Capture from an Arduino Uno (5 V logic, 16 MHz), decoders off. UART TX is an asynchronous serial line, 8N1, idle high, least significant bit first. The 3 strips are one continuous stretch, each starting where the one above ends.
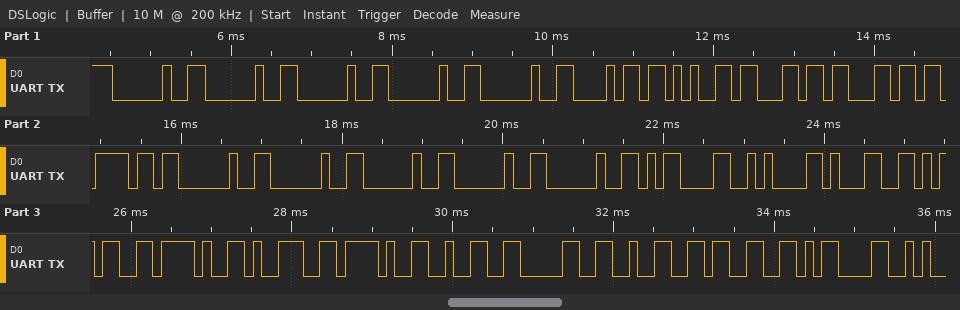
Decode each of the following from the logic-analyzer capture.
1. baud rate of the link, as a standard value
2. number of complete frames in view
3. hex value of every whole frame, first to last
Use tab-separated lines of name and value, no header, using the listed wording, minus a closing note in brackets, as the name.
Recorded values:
baud rate of the link, as a standard value	9600 baud
number of complete frames in view	27
hex value of every whole frame, first to last	0x20 0x20 0x20 0x20 0x20 0x68 0x65 0x6C 0x6C 0x6F 0x20 0x20 0x20 0x20 0x20 0x0D 0x0A 0x31 0x35 0x2F 0x39 0x2F 0x32 0x30 0x32 0x33 0x0D
